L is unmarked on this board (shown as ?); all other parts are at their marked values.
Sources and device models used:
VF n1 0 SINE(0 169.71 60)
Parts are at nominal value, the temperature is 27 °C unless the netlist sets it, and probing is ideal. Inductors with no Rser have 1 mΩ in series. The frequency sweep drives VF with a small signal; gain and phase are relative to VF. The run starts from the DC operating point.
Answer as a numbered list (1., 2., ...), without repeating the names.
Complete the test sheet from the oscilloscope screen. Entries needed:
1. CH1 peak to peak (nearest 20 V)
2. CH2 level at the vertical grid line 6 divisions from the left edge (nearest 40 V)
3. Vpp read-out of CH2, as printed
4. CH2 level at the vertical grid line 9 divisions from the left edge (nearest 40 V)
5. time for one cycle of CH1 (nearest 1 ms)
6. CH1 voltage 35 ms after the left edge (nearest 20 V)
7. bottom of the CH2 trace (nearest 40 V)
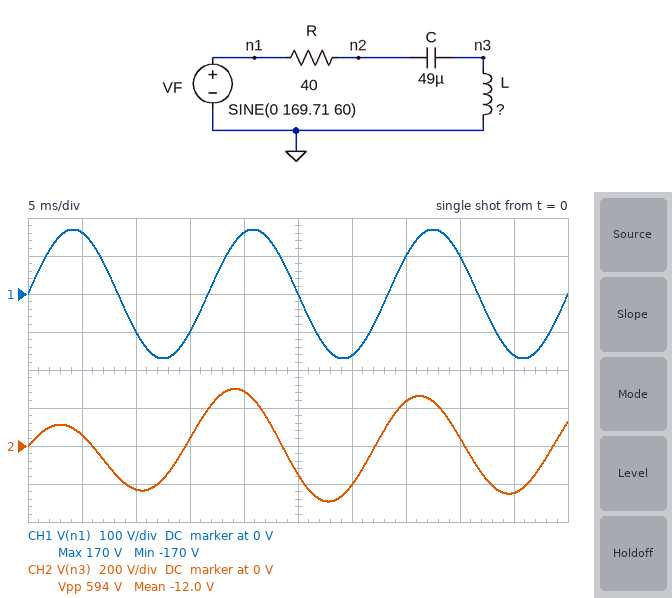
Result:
1. 340 V
2. -200 V
3. 594 V
4. -240 V
5. 17 ms
6. 100 V
7. -280 V
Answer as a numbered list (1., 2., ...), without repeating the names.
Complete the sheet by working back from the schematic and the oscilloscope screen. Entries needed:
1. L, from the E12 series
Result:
1. 330 mH
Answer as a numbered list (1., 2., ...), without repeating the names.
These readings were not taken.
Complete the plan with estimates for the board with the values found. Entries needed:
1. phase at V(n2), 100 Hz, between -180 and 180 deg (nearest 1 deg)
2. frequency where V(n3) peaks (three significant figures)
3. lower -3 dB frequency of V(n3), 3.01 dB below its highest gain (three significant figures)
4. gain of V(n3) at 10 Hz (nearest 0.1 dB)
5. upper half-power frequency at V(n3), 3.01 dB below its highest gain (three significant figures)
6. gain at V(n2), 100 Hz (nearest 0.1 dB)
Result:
1. 13 deg
2. 42.2 Hz
3. 34.0 Hz
4. -23.4 dB
5. 61.9 Hz
6. -0.2 dB
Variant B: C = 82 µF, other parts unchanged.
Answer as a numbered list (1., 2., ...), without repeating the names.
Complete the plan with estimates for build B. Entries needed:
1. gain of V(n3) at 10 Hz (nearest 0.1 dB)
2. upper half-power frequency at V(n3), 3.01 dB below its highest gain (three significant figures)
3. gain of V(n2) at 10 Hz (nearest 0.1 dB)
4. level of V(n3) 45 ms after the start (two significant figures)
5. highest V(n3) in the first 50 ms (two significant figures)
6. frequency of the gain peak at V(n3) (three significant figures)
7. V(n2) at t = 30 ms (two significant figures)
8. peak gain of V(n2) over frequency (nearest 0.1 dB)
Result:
1. -18.7 dB
2. 67.9 Hz
3. -0.2 dB
4. -210 V
5. 240 V
6. 34.2 Hz
7. -130 V
8. 0 dB
